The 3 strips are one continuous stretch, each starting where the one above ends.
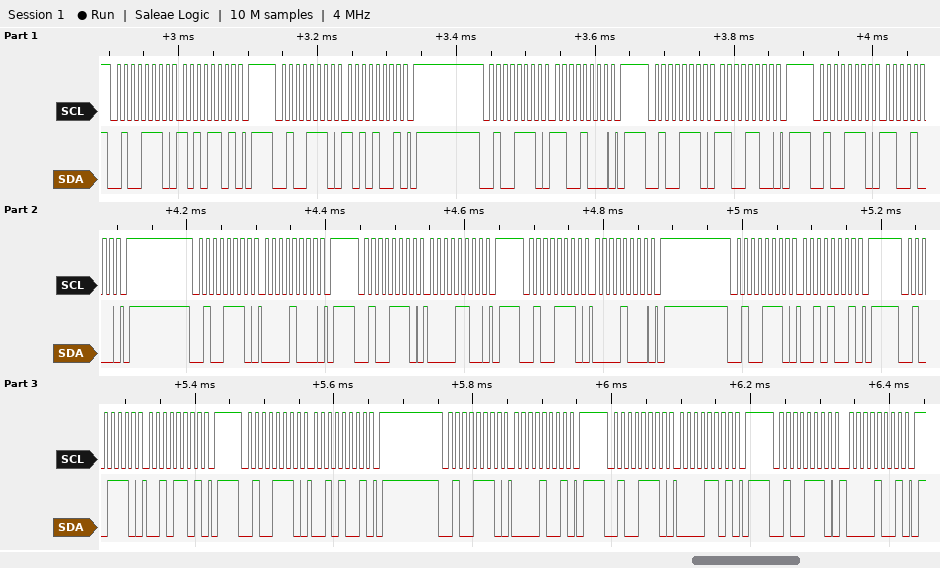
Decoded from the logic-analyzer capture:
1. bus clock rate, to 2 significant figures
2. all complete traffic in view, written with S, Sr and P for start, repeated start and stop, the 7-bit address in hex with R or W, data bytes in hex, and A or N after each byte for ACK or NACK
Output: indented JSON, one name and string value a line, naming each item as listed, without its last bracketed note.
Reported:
{
  "bus clock rate, to 2 significant figures": "100 kHz",
  "all complete traffic in view, written with S, Sr and P for start, repeated start and stop, the 7-bit address in hex with R or W, data bytes in hex, and A or N after each byte for ACK or NACK": "S 27W A AD A P S 27W A A9 A P S 27W A C8 A P S 27W A CC A P S 27W A C8 A P S 27W A 08 A P S 27W A 0C A P S 27W A 08 A P S 27W A 29 A P S 27W A 2D A P S 27W A 29 A P S 27W A 09 A P S 27W A 0D A P S 27W A 09 A P"
}
